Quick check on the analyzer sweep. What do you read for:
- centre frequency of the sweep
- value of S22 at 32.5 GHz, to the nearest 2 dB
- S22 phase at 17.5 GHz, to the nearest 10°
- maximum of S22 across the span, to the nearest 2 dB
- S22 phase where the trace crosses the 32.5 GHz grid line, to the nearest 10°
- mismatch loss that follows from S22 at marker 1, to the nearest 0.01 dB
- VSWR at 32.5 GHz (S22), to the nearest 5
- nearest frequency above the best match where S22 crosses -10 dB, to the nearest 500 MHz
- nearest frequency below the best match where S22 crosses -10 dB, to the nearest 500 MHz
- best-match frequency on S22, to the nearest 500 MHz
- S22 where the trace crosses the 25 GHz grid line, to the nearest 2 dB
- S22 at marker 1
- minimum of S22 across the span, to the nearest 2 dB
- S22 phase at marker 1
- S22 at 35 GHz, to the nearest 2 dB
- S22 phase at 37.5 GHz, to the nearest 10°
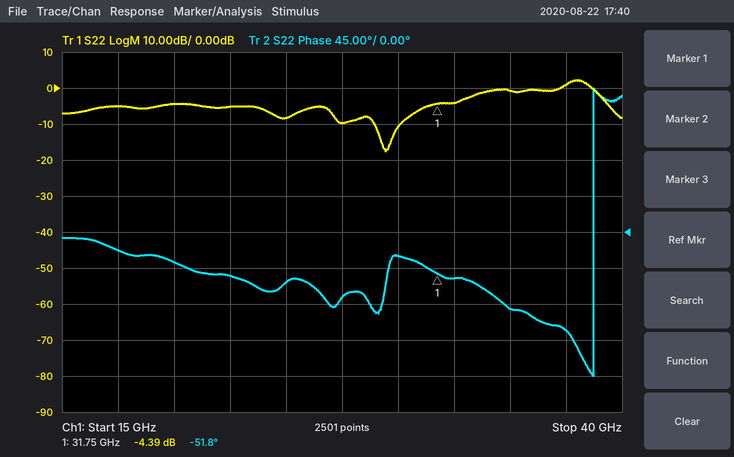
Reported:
27.5 GHz
-4 dB
-20°
2 dB
-60°
1.96 dB
5
30.0 GHz
29.0 GHz
29.5 GHz
-8 dB
-4.39 dB
-18 dB
-51.8°
0 dB
-120°
